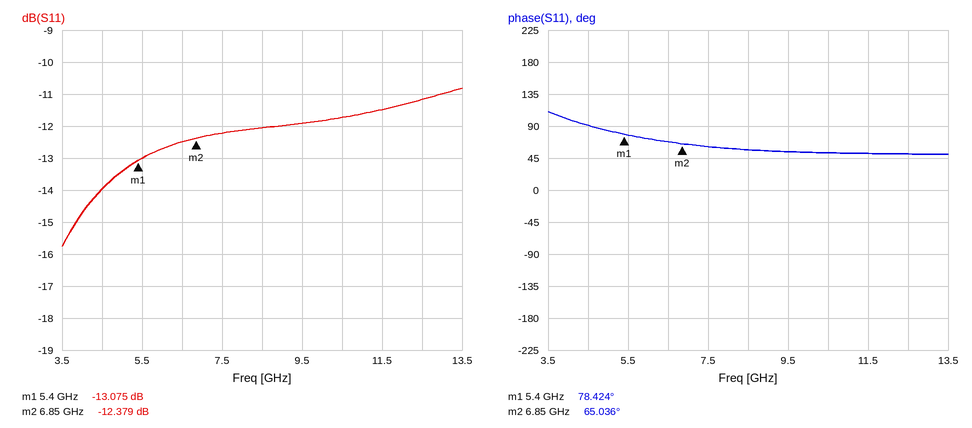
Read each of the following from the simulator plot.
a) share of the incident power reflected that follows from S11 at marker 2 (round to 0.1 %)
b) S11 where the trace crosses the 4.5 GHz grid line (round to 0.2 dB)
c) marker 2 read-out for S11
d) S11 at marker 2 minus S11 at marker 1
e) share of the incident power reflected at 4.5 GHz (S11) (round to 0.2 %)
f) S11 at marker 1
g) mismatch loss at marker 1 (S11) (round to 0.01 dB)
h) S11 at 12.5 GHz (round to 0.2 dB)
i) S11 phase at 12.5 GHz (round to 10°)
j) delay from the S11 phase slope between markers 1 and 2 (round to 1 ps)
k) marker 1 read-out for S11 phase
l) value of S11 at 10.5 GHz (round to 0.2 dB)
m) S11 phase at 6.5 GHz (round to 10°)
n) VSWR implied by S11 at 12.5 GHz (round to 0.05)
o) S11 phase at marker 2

5.8 %
-14.0 dB
-12.379 dB
0.696 dB
4.0 %
-13.075 dB
0.22 dB
-11.2 dB
50°
26 ps
78.424°
-11.8 dB
70°
1.75
65.036°
